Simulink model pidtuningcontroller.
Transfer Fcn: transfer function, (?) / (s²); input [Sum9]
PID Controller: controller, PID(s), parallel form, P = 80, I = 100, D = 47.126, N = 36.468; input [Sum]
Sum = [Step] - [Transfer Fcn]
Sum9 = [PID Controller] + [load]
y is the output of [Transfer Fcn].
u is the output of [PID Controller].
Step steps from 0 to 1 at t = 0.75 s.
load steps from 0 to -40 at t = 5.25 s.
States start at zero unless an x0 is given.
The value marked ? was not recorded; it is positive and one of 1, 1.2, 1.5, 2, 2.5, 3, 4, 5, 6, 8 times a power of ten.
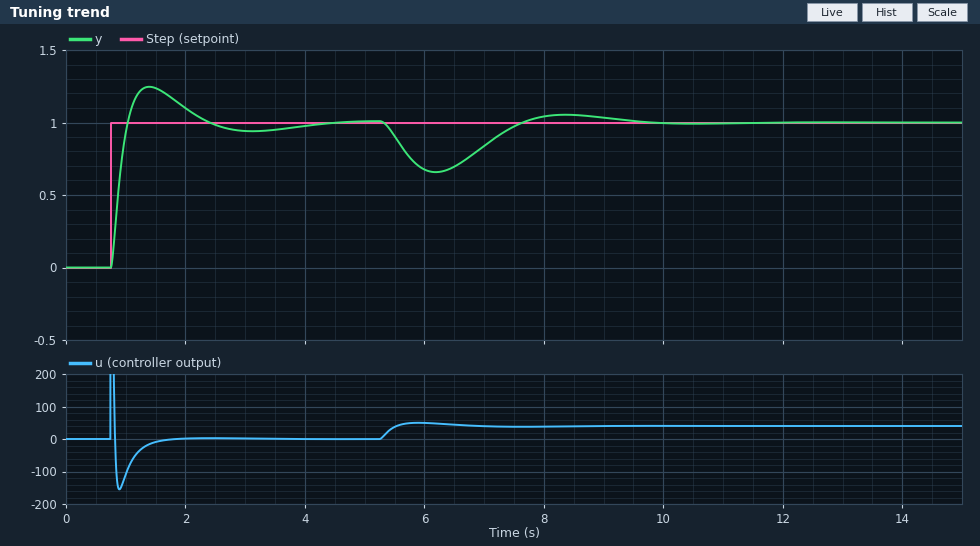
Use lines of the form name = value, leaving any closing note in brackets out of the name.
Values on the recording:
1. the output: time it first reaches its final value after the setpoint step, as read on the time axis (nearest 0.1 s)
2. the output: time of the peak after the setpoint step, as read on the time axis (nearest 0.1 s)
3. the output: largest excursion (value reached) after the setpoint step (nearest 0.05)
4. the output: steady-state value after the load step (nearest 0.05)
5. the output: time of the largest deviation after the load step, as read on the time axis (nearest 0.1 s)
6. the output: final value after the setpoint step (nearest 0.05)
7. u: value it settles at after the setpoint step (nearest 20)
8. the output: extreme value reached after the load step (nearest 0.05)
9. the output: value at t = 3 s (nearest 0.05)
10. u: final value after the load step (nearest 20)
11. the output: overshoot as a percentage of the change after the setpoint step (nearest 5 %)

the output: time it first reaches its final value after the setpoint step, as read on the time axis = 1.0 s
the output: time of the peak after the setpoint step, as read on the time axis = 1.4 s
the output: largest excursion (value reached) after the setpoint step = 1.25
the output: steady-state value after the load step = 1.00
the output: time of the largest deviation after the load step, as read on the time axis = 6.2 s
the output: final value after the setpoint step = 1.00
u: value it settles at after the setpoint step = 0
the output: extreme value reached after the load step = 0.65
the output: value at t = 3 s = 0.95
u: final value after the load step = 40
the output: overshoot as a percentage of the change after the setpoint step = 25 %
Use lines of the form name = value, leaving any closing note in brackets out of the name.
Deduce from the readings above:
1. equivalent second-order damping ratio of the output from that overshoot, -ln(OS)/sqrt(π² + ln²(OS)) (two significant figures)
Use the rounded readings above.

equivalent second-order damping ratio of the output from that overshoot, -ln(OS)/sqrt(π² + ln²(OS)) = 0.40
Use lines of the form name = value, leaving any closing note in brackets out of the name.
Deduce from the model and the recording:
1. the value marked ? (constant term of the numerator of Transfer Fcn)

the value marked ? = 0.12
